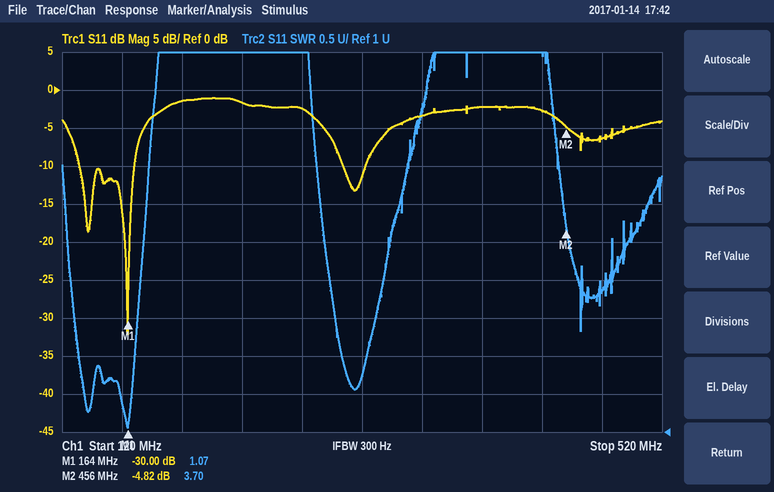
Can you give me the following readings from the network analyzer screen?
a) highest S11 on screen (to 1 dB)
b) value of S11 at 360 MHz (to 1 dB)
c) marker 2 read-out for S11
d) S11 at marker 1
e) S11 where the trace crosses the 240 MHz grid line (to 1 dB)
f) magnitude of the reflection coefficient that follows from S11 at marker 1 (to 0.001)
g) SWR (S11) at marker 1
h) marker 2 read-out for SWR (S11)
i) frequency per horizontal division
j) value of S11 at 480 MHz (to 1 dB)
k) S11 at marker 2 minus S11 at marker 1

-1 dB
-3 dB
-4.82 dB
-30.00 dB
-2 dB
0.032
1.07
3.70
40 MHz
-6 dB
25.18 dB
